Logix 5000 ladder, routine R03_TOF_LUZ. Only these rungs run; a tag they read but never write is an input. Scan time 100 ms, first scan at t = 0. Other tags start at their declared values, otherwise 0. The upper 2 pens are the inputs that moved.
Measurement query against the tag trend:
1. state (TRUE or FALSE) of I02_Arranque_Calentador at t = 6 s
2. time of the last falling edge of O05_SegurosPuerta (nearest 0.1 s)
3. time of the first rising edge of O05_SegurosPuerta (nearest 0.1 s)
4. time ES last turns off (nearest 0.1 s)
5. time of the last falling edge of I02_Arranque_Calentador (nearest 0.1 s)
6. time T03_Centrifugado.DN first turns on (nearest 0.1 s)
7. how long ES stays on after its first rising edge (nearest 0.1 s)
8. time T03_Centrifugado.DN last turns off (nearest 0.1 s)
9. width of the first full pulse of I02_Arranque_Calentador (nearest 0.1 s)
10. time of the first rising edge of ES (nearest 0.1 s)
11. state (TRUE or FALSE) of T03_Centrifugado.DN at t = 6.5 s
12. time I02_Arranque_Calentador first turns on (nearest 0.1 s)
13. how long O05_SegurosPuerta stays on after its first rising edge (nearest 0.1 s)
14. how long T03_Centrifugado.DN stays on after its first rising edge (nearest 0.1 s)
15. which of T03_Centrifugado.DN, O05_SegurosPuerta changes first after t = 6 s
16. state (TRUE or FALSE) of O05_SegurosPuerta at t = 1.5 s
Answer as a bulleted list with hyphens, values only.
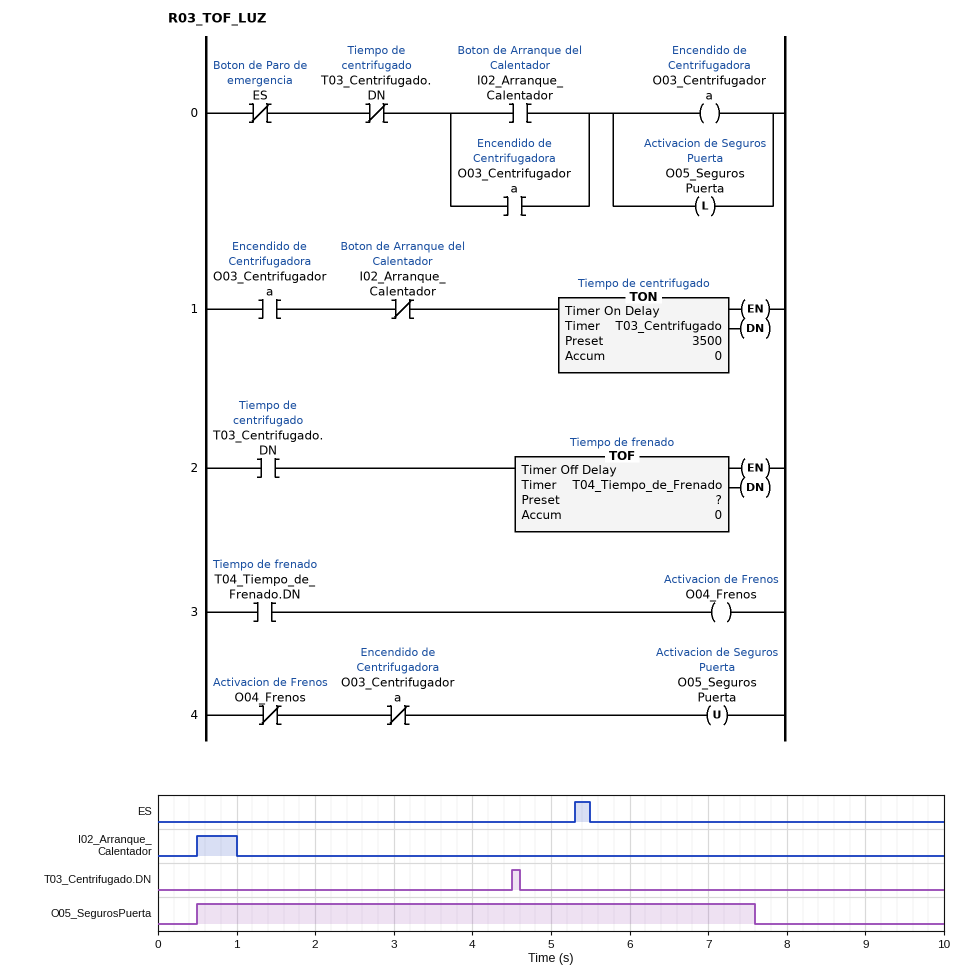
- FALSE
- 7.6 s
- 0.5 s
- 5.5 s
- 1.0 s
- 4.5 s
- 0.2 s
- 4.6 s
- 0.5 s
- 5.3 s
- FALSE
- 0.5 s
- 7.1 s
- 0.1 s
- O05_SegurosPuerta
- TRUE
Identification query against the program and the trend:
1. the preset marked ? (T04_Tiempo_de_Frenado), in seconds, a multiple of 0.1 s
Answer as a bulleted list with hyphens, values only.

- 3.0 s
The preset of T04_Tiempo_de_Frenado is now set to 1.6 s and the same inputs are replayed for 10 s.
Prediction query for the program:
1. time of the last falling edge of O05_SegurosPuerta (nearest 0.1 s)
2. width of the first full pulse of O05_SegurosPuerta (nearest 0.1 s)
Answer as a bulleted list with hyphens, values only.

- 6.2 s
- 5.7 s
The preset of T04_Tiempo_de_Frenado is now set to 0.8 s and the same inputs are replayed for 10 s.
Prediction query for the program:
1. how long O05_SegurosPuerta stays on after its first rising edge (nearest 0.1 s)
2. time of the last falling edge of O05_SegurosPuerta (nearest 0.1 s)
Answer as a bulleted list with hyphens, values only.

- 4.9 s
- 5.4 s
